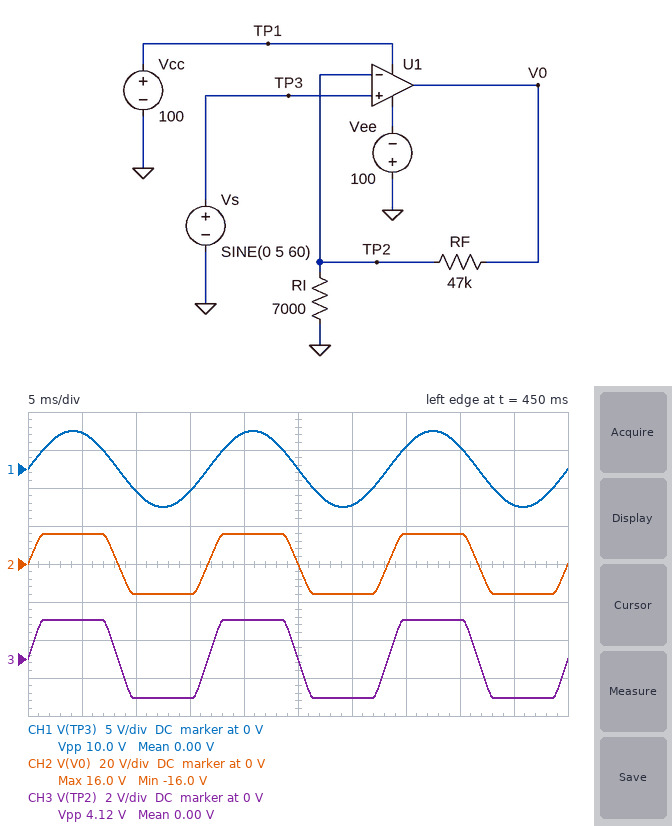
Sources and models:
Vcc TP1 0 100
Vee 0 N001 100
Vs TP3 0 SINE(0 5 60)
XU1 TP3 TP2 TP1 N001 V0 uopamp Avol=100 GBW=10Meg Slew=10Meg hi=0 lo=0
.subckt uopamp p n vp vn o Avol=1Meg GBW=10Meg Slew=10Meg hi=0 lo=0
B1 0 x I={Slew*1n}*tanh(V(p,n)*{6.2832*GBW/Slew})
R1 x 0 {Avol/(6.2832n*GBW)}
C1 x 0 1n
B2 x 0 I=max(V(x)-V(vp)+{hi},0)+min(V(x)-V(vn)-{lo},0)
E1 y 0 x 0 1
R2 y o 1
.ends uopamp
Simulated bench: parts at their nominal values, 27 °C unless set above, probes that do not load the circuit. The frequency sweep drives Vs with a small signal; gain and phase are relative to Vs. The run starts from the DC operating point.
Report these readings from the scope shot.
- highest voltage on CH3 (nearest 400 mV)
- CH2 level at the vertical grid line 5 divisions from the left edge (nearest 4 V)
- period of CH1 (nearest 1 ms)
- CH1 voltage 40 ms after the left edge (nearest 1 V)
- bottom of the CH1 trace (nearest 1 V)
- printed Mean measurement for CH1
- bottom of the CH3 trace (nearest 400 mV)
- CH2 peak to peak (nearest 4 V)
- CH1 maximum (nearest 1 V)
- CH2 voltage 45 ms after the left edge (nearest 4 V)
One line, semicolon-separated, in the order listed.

2.0 V; 0 V; 17 ms; 3 V; -5 V; 0.00 V; -2.0 V; 32 V; 5 V; -16 V
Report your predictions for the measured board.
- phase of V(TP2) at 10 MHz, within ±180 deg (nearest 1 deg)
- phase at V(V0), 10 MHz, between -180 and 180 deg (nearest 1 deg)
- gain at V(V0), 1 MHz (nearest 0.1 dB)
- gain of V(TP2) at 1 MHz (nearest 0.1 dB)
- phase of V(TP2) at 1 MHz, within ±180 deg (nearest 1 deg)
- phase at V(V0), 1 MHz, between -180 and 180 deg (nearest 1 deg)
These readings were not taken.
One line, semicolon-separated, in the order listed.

-82 deg; -82 deg; 15.3 dB; -2.4 dB; -36 deg; -36 deg
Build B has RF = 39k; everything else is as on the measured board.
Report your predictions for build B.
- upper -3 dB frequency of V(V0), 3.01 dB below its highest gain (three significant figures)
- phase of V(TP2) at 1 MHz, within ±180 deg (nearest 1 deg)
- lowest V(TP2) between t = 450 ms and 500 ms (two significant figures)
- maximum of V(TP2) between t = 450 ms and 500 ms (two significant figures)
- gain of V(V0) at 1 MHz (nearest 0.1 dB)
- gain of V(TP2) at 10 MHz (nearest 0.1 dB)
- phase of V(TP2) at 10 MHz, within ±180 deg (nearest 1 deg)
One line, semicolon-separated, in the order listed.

1.62 MHz; -32 deg; -2.4 V; 2.4 V; 14.4 dB; -16.5 dB; -81 deg
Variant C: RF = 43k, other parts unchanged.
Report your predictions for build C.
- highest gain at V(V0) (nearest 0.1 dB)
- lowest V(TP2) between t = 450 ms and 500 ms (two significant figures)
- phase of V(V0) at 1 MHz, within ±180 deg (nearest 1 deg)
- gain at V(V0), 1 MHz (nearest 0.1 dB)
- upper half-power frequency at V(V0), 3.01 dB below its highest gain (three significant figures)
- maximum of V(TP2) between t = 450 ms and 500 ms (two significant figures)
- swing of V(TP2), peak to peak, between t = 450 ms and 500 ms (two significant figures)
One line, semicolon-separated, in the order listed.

16.5 dB; -2.2 V; -34 deg; 14.9 dB; 1.50 MHz; 2.2 V; 4.5 V
